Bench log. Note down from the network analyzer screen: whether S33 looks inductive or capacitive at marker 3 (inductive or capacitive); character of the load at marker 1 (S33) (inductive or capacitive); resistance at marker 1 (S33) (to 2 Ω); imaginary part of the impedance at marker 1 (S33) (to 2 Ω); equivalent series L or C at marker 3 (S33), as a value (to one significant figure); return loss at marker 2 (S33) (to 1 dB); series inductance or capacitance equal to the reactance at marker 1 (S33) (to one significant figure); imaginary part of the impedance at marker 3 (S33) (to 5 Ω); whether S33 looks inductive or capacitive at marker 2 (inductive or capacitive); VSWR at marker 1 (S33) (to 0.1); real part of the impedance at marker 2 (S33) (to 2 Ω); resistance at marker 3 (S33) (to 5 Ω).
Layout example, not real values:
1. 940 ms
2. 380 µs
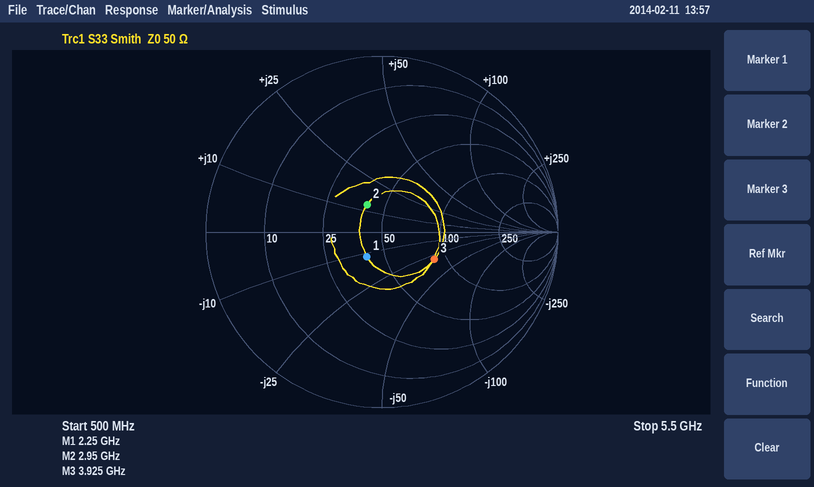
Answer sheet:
1. capacitive
2. capacitive
3. 40 Ω
4. -12 Ω
5. 1 pF
6. 15 dB
7. 6 pF
8. -30 Ω
9. inductive
10. 1.4
11. 40 Ω
12. 85 Ω
